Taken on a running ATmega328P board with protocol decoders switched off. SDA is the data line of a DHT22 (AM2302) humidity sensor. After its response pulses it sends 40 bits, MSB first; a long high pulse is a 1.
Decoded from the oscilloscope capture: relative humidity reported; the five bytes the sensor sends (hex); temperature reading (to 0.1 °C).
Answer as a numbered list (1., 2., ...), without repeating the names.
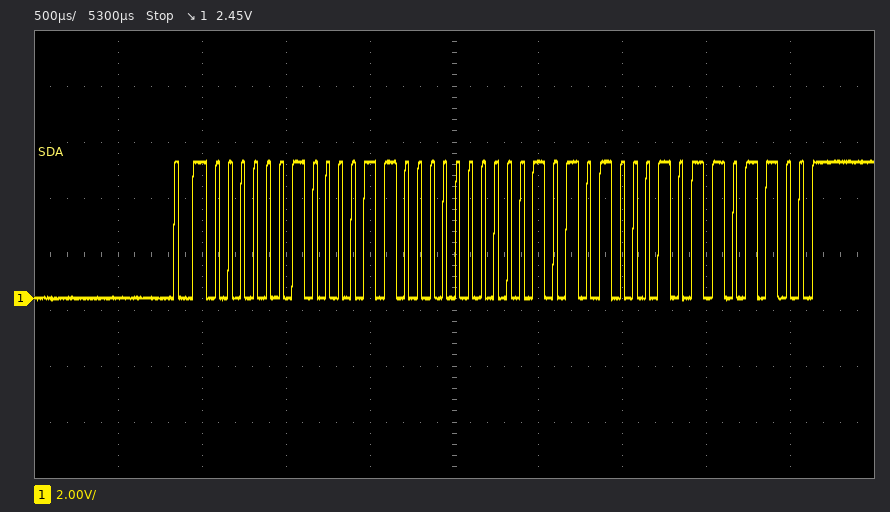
1. 53.6 %
2. 02 18 01 51 6C
3. 33.7 °C
